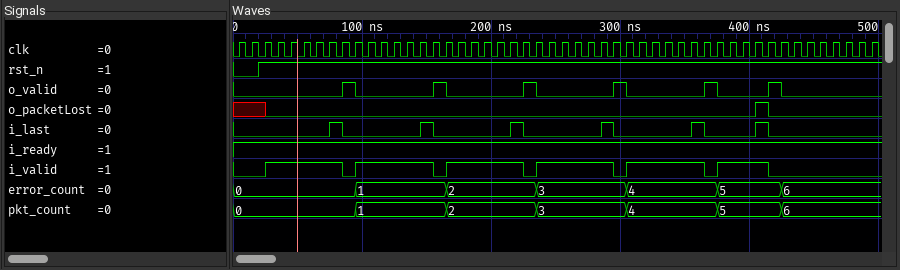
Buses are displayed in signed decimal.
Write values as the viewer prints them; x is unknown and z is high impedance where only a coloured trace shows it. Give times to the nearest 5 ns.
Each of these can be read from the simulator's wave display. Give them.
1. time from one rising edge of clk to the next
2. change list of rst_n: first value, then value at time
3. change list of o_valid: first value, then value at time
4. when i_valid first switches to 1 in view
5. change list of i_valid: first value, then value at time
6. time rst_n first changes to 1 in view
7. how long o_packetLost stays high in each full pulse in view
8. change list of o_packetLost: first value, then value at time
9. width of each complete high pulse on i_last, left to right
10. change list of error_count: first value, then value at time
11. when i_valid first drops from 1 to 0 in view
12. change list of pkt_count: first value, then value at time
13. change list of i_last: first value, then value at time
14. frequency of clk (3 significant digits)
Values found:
10 ns
0, 1 at 20 ns
0, 1 at 85 ns, 0 at 95 ns, 1 at 155 ns, 0 at 165 ns, 1 at 225 ns, 0 at 235 ns, 1 at 295 ns, 0 at 305 ns, 1 at 365 ns, 0 at 375 ns, 1 at 415 ns, 0 at 425 ns
25 ns
0, 1 at 25 ns, 0 at 85 ns, 1 at 95 ns, 0 at 155 ns, 1 at 165 ns, 0 at 225 ns, 1 at 235 ns, 0 at 295 ns, 1 at 305 ns, 0 at 365 ns, 1 at 375 ns, 0 at 415 ns
20 ns
10 ns
x, 0 at 25 ns, 1 at 405 ns, 0 at 415 ns
10 ns, 10 ns, 10 ns, 10 ns, 10 ns, 10 ns
0, 1 at 95 ns, 2 at 165 ns, 3 at 235 ns, 4 at 305 ns, 5 at 375 ns, 6 at 425 ns
85 ns
0, 1 at 95 ns, 2 at 165 ns, 3 at 235 ns, 4 at 305 ns, 5 at 375 ns, 6 at 425 ns
0, 1 at 75 ns, 0 at 85 ns, 1 at 145 ns, 0 at 155 ns, 1 at 215 ns, 0 at 225 ns, 1 at 285 ns, 0 at 295 ns, 1 at 355 ns, 0 at 365 ns, 1 at 405 ns, 0 at 415 ns
100 MHz
